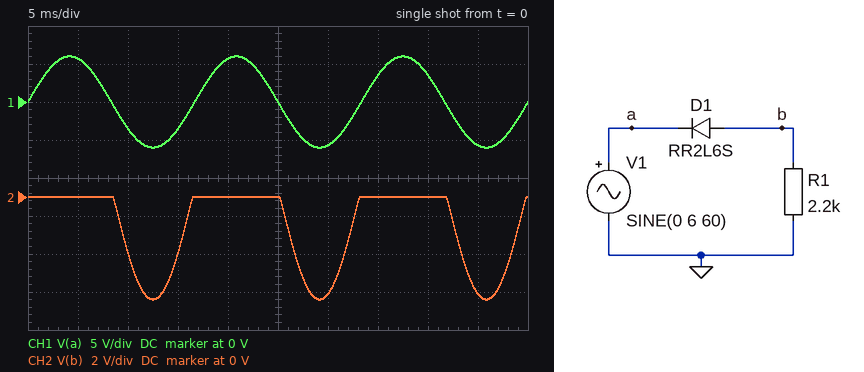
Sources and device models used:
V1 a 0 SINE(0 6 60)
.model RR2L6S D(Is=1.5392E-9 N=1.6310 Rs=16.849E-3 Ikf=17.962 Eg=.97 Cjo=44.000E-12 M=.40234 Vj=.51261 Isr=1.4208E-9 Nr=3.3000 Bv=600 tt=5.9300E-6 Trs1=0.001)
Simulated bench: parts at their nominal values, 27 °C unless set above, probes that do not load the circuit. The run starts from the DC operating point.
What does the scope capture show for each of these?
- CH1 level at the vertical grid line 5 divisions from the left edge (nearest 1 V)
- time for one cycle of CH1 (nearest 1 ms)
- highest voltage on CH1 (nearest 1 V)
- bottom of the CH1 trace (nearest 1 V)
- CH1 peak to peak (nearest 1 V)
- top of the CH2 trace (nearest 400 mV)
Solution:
0 V
17 ms
6 V
-6 V
12 V
0 V
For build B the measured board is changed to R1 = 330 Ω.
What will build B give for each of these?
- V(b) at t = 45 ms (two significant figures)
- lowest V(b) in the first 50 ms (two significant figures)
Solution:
-5.0 V
-5.3 V
